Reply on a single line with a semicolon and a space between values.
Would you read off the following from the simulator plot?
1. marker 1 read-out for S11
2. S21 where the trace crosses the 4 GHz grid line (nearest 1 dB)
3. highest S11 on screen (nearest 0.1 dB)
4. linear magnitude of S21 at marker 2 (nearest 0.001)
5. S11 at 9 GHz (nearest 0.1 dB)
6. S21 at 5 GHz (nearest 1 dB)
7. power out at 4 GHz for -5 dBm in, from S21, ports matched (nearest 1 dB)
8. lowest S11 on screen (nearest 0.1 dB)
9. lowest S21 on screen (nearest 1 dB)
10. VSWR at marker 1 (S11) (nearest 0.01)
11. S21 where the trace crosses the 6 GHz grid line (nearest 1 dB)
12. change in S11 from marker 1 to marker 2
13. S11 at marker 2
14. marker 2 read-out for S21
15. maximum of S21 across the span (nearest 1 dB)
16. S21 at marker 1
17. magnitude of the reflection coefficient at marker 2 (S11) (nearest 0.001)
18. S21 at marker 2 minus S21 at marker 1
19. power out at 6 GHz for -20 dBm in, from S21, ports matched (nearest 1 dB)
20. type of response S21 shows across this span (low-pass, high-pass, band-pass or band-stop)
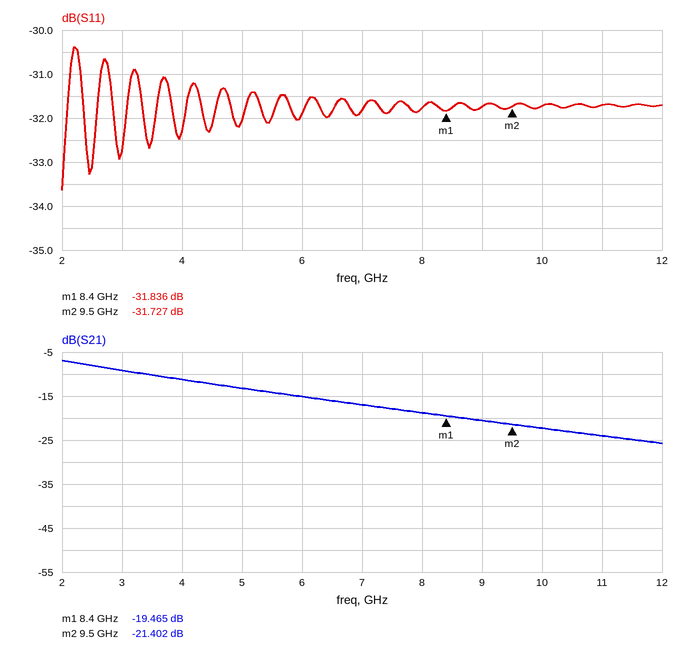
-31.836 dB; -11 dB; -30.4 dB; 0.085; -31.7 dB; -13 dB; -16 dBm; -33.6 dB; -26 dB; 1.05; -15 dB; 0.109 dB; -31.727 dB; -21.402 dB; -7 dB; -19.465 dB; 0.026; -1.937 dB; -35 dBm; low-pass
